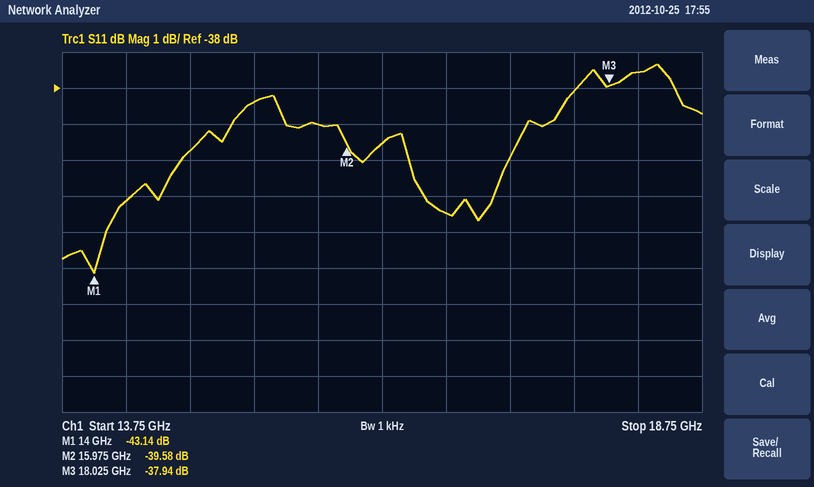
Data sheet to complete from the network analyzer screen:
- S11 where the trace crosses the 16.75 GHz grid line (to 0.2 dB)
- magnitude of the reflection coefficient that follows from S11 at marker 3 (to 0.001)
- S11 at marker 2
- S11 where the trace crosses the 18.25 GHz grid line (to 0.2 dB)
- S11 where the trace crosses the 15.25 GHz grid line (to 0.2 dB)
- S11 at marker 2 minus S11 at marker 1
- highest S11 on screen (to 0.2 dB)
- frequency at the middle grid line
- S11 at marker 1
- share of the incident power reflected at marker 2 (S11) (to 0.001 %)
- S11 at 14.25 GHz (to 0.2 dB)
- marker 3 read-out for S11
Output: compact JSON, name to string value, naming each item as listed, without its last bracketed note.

{"S11 where the trace crosses the 16.75 GHz grid line": "-41.4 dB", "magnitude of the reflection coefficient that follows from S11 at marker 3": "0.013", "S11 at marker 2": "-39.58 dB", "S11 where the trace crosses the 18.25 GHz grid line": "-37.6 dB", "S11 where the trace crosses the 15.25 GHz grid line": "-38.4 dB", "S11 at marker 2 minus S11 at marker 1": "3.56 dB", "highest S11 on screen": "-37.4 dB", "frequency at the middle grid line": "16.25 GHz", "S11 at marker 1": "-43.14 dB", "share of the incident power reflected at marker 2 (S11)": "0.011 %", "S11 at 14.25 GHz": "-41.2 dB", "marker 3 read-out for S11": "-37.94 dB"}
